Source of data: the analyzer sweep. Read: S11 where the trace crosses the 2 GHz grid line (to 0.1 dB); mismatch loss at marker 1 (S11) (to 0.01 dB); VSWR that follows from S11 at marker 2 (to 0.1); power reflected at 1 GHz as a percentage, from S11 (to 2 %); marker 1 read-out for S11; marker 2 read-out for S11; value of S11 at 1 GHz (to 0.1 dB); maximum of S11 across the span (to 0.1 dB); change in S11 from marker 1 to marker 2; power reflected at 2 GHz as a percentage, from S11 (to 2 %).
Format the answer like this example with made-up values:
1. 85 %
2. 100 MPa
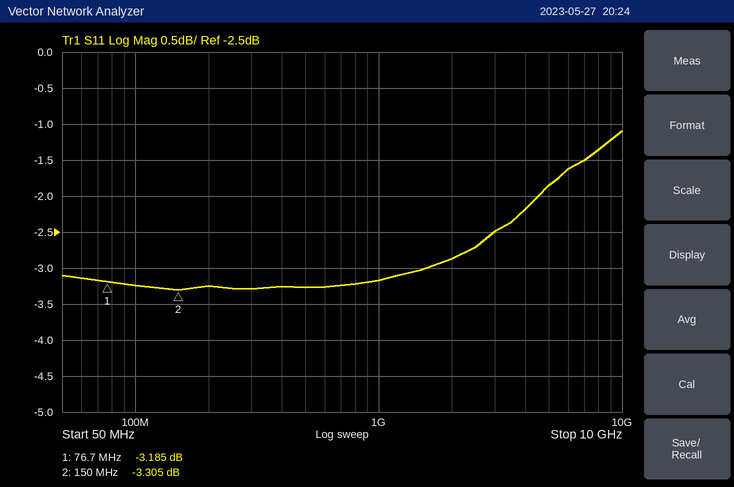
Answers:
1. -2.9 dB
2. 2.84 dB
3. 5.3
4. 48 %
5. -3.185 dB
6. -3.305 dB
7. -3.2 dB
8. -1.1 dB
9. -0.120 dB
10. 52 %
